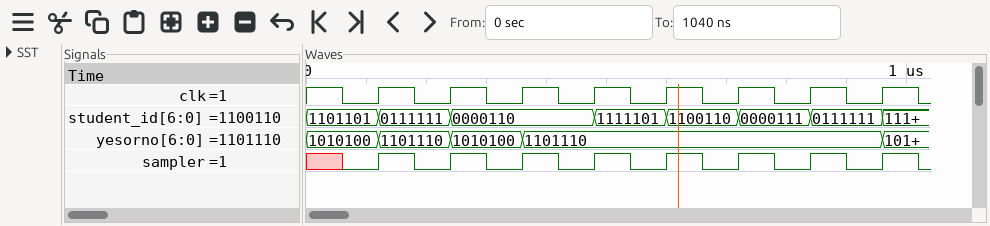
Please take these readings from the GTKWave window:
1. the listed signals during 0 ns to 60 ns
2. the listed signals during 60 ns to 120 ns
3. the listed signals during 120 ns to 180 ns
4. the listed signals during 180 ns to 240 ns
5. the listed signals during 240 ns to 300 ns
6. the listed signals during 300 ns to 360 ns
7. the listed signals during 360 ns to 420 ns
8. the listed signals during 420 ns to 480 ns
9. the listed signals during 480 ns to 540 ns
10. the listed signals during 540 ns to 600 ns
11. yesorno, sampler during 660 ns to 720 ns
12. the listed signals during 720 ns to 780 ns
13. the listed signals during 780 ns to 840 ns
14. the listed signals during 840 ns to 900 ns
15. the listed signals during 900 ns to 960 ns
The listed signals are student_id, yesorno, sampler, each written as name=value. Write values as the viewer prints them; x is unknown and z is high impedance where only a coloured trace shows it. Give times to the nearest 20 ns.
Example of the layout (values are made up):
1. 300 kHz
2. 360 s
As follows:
1. student_id=1101101, yesorno=1010100, sampler=x
2. student_id=1101101, yesorno=1010100, sampler=0
3. student_id=0111111, yesorno=1101110, sampler=1
4. student_id=0111111, yesorno=1101110, sampler=0
5. student_id=0000110, yesorno=1010100, sampler=1
6. student_id=0000110, yesorno=1010100, sampler=0
7. student_id=0000110, yesorno=1101110, sampler=1
8. student_id=0000110, yesorno=1101110, sampler=0
9. student_id=1111101, yesorno=1101110, sampler=1
10. student_id=1111101, yesorno=1101110, sampler=0
11. yesorno=1101110, sampler=0
12. student_id=0000111, yesorno=1101110, sampler=1
13. student_id=0000111, yesorno=1101110, sampler=0
14. student_id=0111111, yesorno=1101110, sampler=1
15. student_id=0111111, yesorno=1101110, sampler=0
